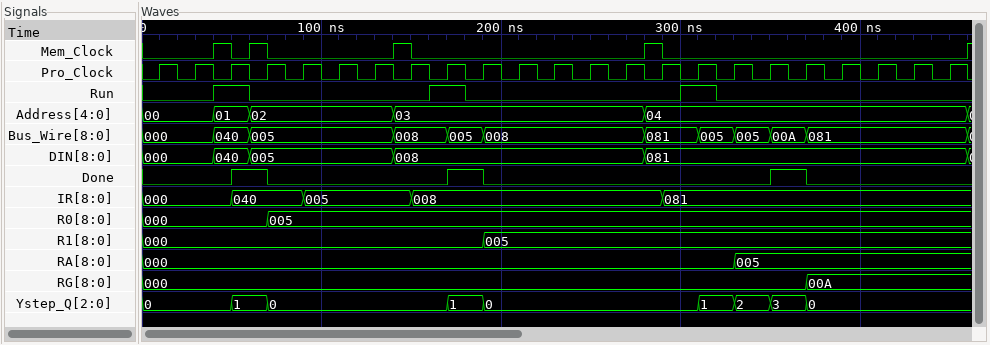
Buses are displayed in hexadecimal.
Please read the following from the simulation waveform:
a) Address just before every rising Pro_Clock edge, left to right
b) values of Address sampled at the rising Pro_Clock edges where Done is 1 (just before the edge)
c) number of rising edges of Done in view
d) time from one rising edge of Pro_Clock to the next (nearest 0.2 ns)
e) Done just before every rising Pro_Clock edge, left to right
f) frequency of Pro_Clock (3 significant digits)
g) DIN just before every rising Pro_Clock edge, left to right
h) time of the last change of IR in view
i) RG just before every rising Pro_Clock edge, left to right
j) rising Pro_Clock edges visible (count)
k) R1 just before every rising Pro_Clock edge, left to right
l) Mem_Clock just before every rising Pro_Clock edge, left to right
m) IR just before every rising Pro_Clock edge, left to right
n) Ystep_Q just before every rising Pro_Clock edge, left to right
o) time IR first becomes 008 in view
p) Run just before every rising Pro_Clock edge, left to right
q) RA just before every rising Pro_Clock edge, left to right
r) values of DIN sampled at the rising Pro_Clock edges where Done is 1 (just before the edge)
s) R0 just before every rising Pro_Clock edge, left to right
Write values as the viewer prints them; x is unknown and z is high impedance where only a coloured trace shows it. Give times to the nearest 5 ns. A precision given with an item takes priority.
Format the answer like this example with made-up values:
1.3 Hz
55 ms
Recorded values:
00, 00, 01, 02, 02, 02, 02, 03, 03, 03, 03, 03, 03, 03, 04, 04, 04, 04, 04, 04, 04, 04, 04
02, 03, 04
3
20 ns
0 0 0 1 0 0 0 0 0 1 0 0 0 0 0 0 0 0 1 0 0 0 0
50.0 MHz
000, 000, 040, 005, 005, 005, 005, 008, 008, 008, 008, 008, 008, 008, 081, 081, 081, 081, 081, 081, 081, 081, 081
290 ns
000, 000, 000, 000, 000, 000, 000, 000, 000, 000, 000, 000, 000, 000, 000, 000, 000, 000, 000, 00A, 00A, 00A, 00A
23
000, 000, 000, 000, 000, 000, 000, 000, 000, 000, 005, 005, 005, 005, 005, 005, 005, 005, 005, 005, 005, 005, 005
0 0 1 1 0 0 0 1 0 0 0 0 0 0 1 0 0 0 0 0 0 0 0
000, 000, 000, 040, 040, 005, 005, 005, 008, 008, 008, 008, 008, 008, 008, 081, 081, 081, 081, 081, 081, 081, 081
0, 0, 0, 1, 0, 0, 0, 0, 0, 1, 0, 0, 0, 0, 0, 0, 1, 2, 3, 0, 0, 0, 0
150 ns
0 0 1 0 0 0 0 0 1 0 0 0 0 0 0 1 0 0 0 0 0 0 0
000, 000, 000, 000, 000, 000, 000, 000, 000, 000, 000, 000, 000, 000, 000, 000, 000, 005, 005, 005, 005, 005, 005
005, 008, 081
000, 000, 000, 000, 005, 005, 005, 005, 005, 005, 005, 005, 005, 005, 005, 005, 005, 005, 005, 005, 005, 005, 005
